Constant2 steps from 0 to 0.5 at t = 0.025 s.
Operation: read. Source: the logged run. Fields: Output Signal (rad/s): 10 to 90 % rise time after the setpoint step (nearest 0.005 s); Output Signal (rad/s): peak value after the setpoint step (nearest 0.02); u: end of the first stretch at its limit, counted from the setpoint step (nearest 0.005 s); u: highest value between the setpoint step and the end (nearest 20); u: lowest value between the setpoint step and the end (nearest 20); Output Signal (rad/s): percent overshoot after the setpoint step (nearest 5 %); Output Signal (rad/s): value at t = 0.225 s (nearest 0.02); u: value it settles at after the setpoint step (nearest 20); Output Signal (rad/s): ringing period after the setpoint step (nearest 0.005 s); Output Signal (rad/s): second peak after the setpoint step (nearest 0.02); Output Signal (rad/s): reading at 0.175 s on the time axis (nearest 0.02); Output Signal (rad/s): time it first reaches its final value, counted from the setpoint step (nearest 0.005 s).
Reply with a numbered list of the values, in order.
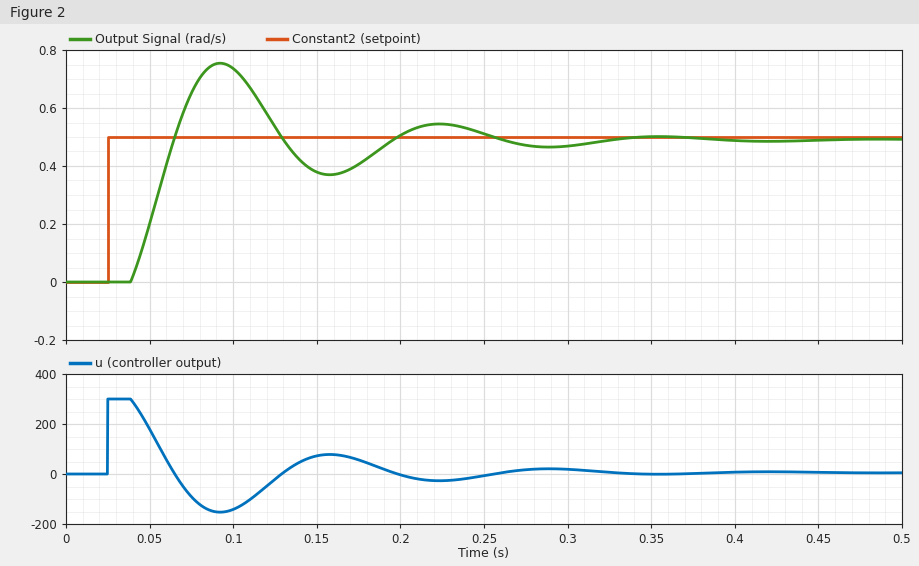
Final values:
1. 0.020 s
2. 0.76
3. 0.015 s
4. 300
5. -160
6. 55 %
7. 0.54
8. 0
9. 0.130 s
10. 0.54
11. 0.40
12. 0.040 s
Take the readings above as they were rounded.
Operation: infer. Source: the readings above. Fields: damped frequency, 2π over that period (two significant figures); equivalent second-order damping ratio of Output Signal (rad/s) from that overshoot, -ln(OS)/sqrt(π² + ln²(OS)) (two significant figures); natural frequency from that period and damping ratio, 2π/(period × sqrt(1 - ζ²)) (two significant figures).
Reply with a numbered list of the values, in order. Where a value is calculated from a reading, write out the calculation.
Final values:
1. 2π / 0.13 = 48 rad/s
2. ln(0.55) = -0.598; 0.598 / sqrt(9.870 + 0.357) = 0.19
3. 2π / (0.13 × sqrt(1 - 0.19²)) = 49 rad/s
